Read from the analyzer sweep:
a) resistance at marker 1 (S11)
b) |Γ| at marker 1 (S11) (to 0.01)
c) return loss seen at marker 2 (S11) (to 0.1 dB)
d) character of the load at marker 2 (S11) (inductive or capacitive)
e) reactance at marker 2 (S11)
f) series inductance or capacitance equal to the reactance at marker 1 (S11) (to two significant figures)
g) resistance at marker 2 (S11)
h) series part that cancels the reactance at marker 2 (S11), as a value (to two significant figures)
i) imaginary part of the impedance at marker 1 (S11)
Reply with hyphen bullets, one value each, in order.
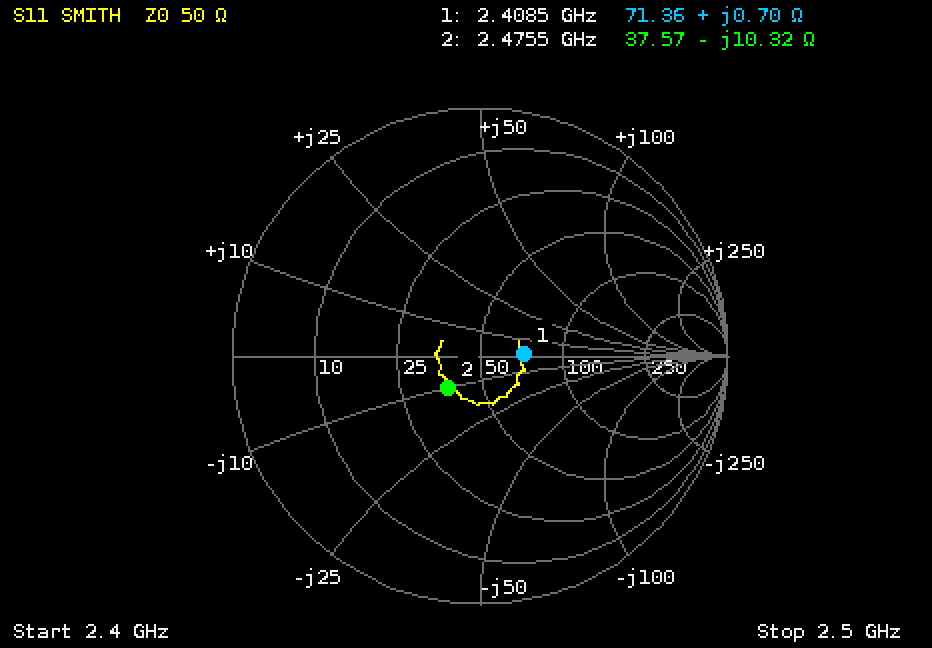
- 71.36 Ω
- 0.18
- 14.7 dB
- capacitive
- -10.32 Ω
- 46 pH
- 37.57 Ω
- 660 pH
- +0.70 Ω
